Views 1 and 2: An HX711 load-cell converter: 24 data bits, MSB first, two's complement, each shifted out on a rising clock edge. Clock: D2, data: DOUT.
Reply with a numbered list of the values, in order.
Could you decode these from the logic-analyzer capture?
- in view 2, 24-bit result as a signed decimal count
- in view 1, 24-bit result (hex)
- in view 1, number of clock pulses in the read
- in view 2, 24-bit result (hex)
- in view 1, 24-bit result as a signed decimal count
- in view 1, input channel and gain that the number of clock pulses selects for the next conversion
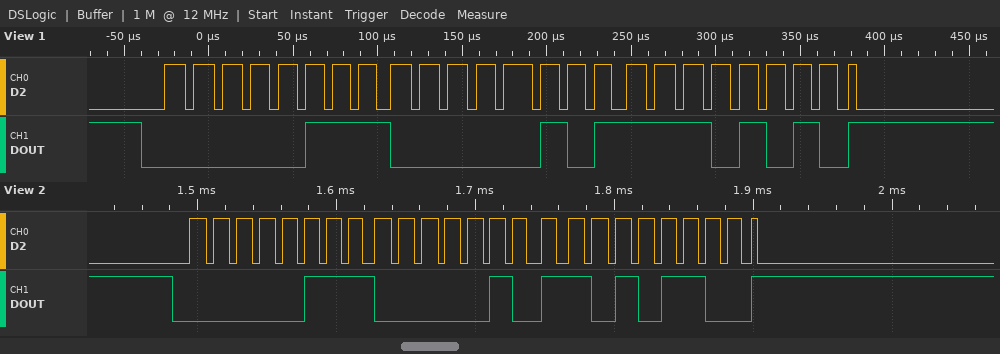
1. 460204
2. 0x0705EA
3. 25
4. 0x0705AC
5. 460266
6. channel A, gain 128
